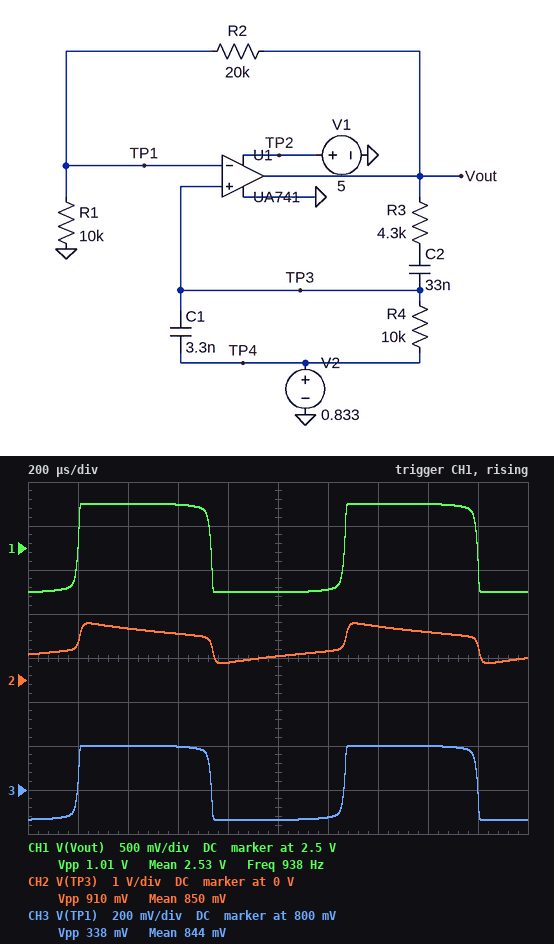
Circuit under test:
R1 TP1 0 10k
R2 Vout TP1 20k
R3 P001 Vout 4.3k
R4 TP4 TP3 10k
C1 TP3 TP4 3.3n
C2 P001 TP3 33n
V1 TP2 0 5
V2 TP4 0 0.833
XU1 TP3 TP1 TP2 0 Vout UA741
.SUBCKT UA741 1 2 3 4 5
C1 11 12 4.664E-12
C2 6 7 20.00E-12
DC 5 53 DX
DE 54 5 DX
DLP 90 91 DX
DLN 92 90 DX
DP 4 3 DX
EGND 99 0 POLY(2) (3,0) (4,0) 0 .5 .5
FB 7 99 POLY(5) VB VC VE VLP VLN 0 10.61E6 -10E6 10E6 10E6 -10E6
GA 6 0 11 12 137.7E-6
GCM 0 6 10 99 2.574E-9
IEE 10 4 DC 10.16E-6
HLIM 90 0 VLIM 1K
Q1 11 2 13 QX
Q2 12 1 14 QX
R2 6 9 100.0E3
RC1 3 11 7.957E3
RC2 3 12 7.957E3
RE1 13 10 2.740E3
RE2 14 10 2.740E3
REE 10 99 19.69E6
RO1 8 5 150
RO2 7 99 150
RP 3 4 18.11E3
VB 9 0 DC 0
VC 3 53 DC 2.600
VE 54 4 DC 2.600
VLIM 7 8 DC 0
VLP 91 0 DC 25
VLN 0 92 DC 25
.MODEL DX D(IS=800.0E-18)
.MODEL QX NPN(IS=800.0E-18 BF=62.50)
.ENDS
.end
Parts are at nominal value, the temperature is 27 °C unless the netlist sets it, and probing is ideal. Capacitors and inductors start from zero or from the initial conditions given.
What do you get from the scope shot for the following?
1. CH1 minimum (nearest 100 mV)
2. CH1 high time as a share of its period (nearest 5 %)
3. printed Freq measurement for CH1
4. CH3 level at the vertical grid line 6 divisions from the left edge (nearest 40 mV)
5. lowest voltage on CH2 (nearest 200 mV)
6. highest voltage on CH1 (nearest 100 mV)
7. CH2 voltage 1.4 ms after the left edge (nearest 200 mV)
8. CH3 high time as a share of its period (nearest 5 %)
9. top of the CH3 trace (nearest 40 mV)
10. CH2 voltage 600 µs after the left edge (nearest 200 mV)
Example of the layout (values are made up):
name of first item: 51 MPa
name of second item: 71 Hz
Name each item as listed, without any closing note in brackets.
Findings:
CH1 minimum: 2.0 V
CH1 high time as a share of its period: 50 %
printed Freq measurement for CH1: 938 Hz
CH3 level at the vertical grid line 6 divisions from the left edge: 680 mV
lowest voltage on CH2: 400 mV
highest voltage on CH1: 3.0 V
CH2 voltage 1.4 ms after the left edge: 1.2 V
CH3 high time as a share of its period: 50 %
top of the CH3 trace: 1.00 V
CH2 voltage 600 µs after the left edge: 1.0 V
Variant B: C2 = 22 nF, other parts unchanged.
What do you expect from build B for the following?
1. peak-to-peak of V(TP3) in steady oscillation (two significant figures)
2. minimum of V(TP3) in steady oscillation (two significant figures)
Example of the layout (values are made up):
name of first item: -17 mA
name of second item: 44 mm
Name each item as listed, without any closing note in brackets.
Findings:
peak-to-peak of V(TP3) in steady oscillation: 870 mV
minimum of V(TP3) in steady oscillation: 400 mV
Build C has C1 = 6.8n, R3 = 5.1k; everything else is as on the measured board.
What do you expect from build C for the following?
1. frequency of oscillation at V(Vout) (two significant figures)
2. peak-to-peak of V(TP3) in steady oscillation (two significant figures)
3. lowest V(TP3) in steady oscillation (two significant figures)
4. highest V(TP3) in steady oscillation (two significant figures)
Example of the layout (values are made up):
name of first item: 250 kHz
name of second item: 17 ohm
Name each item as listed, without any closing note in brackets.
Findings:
frequency of oscillation at V(Vout): 850 Hz
peak-to-peak of V(TP3) in steady oscillation: 770 mV
lowest V(TP3) in steady oscillation: 450 mV
highest V(TP3) in steady oscillation: 1.2 V
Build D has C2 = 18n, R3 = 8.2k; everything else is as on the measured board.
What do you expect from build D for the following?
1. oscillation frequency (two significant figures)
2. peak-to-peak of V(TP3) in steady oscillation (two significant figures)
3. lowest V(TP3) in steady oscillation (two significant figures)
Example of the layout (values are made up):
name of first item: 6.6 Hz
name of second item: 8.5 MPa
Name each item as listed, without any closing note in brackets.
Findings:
oscillation frequency: 1.5 kHz
peak-to-peak of V(TP3) in steady oscillation: 630 mV
lowest V(TP3) in steady oscillation: 520 mV
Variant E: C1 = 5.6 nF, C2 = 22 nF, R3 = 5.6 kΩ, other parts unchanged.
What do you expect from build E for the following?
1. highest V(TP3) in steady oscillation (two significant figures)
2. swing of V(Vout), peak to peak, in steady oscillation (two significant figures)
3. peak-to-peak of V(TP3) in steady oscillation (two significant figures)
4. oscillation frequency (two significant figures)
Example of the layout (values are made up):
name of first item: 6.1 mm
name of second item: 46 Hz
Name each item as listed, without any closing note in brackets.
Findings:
highest V(TP3) in steady oscillation: 1.2 V
swing of V(Vout), peak to peak, in steady oscillation: 1.0 V
peak-to-peak of V(TP3) in steady oscillation: 710 mV
oscillation frequency: 1.2 kHz
